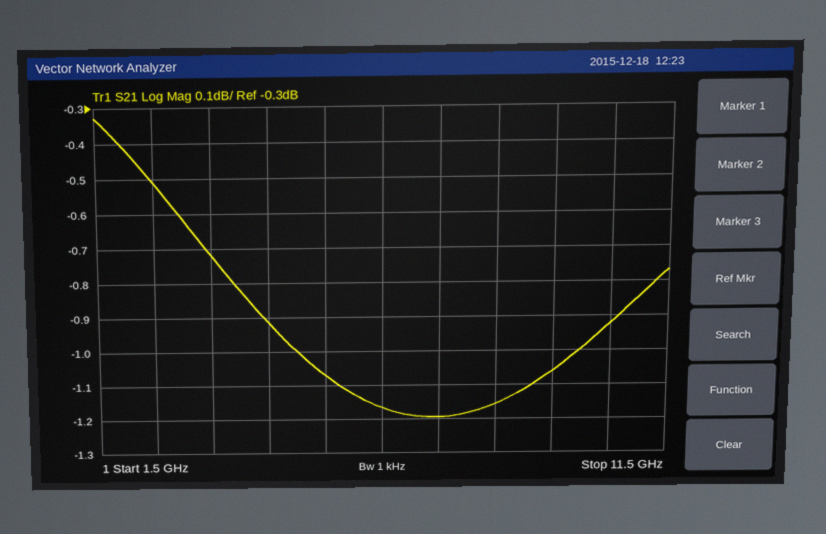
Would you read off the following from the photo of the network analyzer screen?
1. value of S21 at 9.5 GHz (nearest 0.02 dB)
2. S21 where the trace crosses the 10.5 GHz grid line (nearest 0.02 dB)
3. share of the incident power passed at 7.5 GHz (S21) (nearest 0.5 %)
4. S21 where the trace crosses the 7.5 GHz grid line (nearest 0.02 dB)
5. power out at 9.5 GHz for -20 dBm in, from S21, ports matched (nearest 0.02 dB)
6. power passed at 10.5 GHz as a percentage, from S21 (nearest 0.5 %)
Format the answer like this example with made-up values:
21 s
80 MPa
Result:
-1.06 dB
-0.92 dB
76.0 %
-1.20 dB
-21.06 dBm
81.0 %
